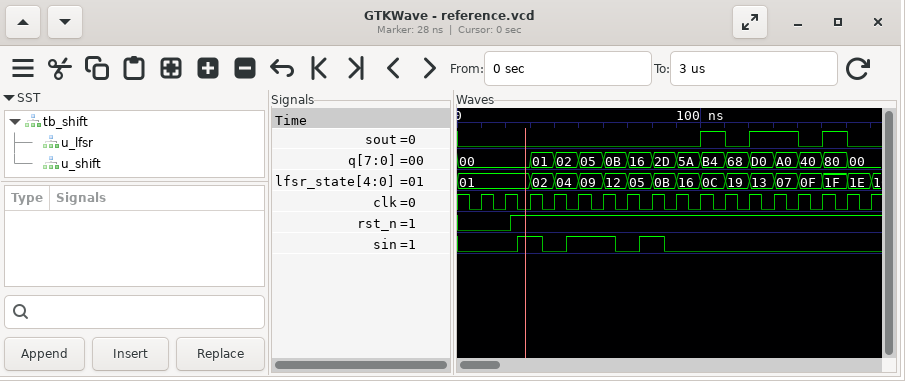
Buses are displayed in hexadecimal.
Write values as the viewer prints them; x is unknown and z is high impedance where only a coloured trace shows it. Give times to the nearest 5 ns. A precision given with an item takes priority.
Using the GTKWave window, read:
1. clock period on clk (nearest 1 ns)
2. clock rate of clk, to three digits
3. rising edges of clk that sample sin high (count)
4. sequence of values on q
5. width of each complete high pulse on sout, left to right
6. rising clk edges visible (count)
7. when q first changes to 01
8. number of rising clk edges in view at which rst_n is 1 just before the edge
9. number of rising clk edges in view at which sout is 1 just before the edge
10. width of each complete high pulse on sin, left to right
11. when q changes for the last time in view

10 ns
100 MHz
4
00, 01, 02, 05, 0B, 16, 2D, 5A, B4, 68, D0, A0, 40, 80, 00
10 ns, 20 ns, 10 ns
17
30 ns
15
4
10 ns, 20 ns, 10 ns
160 ns
